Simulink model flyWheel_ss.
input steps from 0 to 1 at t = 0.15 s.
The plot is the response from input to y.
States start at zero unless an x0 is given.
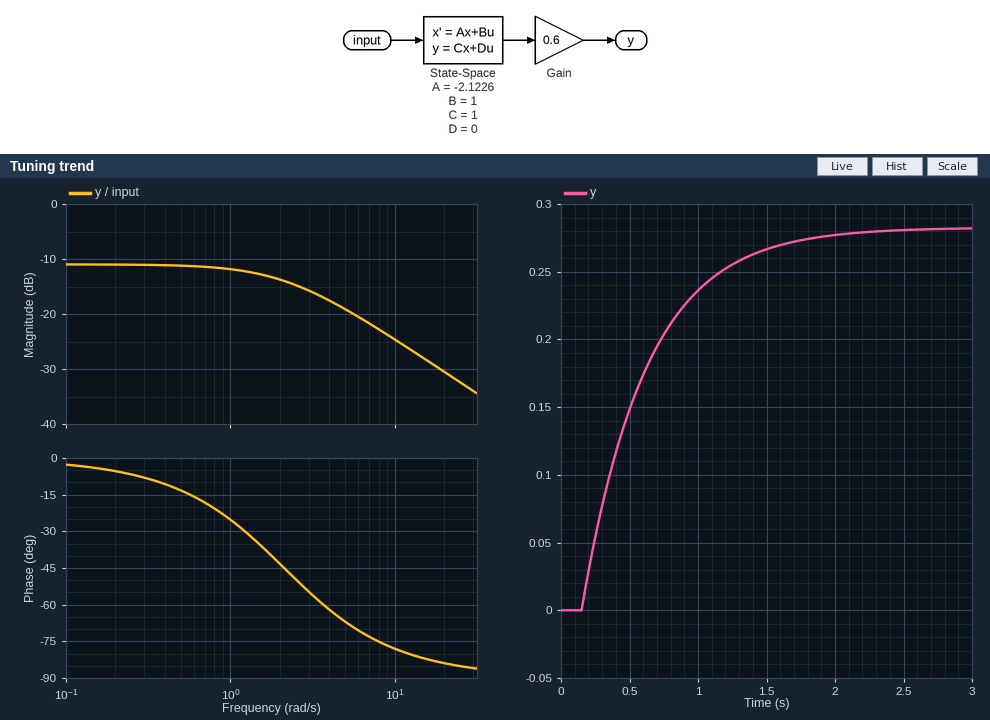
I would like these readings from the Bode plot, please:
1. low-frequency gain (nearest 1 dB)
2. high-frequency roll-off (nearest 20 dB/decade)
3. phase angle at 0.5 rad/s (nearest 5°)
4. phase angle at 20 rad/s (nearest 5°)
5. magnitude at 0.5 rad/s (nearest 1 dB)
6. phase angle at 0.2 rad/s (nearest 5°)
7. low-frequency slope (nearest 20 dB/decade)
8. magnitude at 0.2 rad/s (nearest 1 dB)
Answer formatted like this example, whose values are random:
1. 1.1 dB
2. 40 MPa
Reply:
1. -11 dB
2. -20 dB/decade
3. -15°
4. -85°
5. -11 dB
6. -5°
7. 0 dB/decade
8. -11 dB
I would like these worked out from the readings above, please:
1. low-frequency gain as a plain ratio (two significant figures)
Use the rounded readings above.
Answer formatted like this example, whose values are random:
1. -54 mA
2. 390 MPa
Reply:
1. 0.28
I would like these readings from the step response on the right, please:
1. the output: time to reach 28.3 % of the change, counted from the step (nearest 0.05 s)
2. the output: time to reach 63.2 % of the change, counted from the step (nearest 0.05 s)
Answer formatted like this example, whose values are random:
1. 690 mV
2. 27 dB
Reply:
1. 0.15 s
2. 0.45 s
